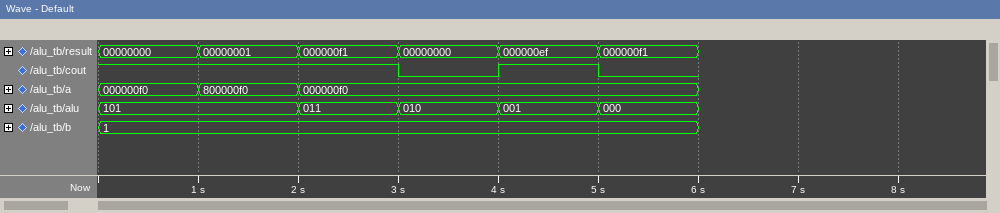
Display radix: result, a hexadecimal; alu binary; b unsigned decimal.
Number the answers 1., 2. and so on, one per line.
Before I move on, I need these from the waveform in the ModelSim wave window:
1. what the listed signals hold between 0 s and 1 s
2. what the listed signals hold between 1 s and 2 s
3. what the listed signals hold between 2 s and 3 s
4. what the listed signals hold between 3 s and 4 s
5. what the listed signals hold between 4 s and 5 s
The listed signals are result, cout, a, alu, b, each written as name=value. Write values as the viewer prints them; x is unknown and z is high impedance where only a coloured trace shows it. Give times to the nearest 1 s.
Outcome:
1. result=00000000, cout=1, a=000000f0, alu=101, b=1
2. result=00000001, cout=1, a=800000f0, alu=101, b=1
3. result=000000f1, cout=1, a=000000f0, alu=011, b=1
4. result=00000000, cout=0, a=000000f0, alu=010, b=1
5. result=000000ef, cout=1, a=000000f0, alu=001, b=1
